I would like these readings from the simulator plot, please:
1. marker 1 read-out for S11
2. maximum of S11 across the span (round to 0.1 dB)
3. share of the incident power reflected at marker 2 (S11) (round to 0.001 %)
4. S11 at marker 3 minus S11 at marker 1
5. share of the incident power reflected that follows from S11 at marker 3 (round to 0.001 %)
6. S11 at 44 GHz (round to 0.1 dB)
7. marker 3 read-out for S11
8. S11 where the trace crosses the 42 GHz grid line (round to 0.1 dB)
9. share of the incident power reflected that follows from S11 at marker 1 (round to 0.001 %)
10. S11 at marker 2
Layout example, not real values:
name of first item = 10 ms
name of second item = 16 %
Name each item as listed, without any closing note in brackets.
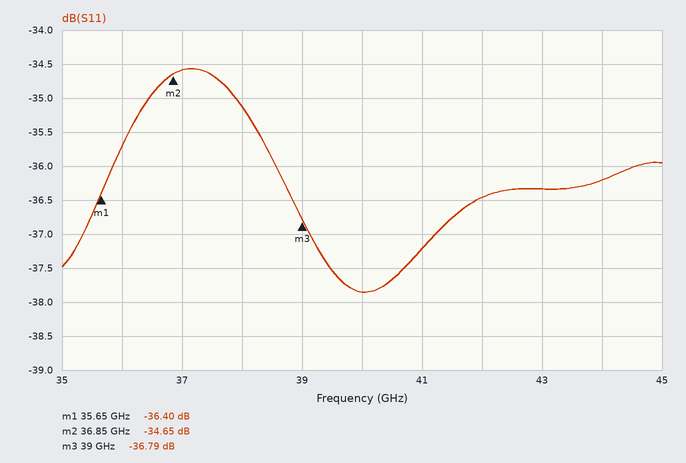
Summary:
marker 1 read-out for S11 = -36.40 dB
maximum of S11 across the span = -34.6 dB
share of the incident power reflected at marker 2 (S11) = 0.034 %
S11 at marker 3 minus S11 at marker 1 = -0.39 dB
share of the incident power reflected that follows from S11 at marker 3 = 0.021 %
S11 at 44 GHz = -36.2 dB
marker 3 read-out for S11 = -36.79 dB
S11 where the trace crosses the 42 GHz grid line = -36.5 dB
share of the incident power reflected that follows from S11 at marker 1 = 0.023 %
S11 at marker 2 = -34.65 dB
